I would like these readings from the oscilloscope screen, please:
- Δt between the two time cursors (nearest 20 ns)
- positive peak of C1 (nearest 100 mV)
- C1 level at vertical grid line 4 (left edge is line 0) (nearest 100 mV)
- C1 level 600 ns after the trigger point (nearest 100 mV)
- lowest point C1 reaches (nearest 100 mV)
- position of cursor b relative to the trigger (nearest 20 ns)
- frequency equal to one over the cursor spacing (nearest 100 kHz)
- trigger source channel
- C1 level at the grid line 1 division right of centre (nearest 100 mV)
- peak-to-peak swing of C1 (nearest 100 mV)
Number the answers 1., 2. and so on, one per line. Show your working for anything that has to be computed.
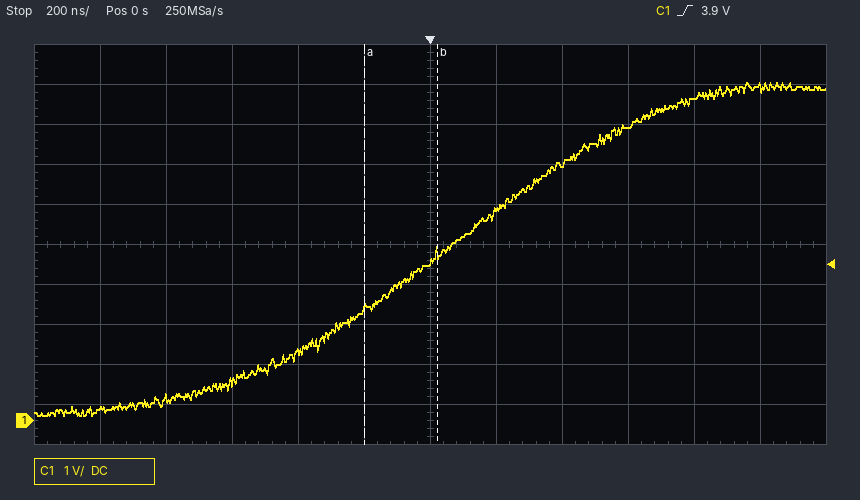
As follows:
1. 220 ns
2. 8.4 V
3. 1.7 V
4. 7.3 V
5. 100 mV
6. +20 ns
7. 1 / 220 ns ≈ 4.5 MHz
8. C1
9. 5.2 V
10. 8.4 V − (100 mV) = 8.3 V
